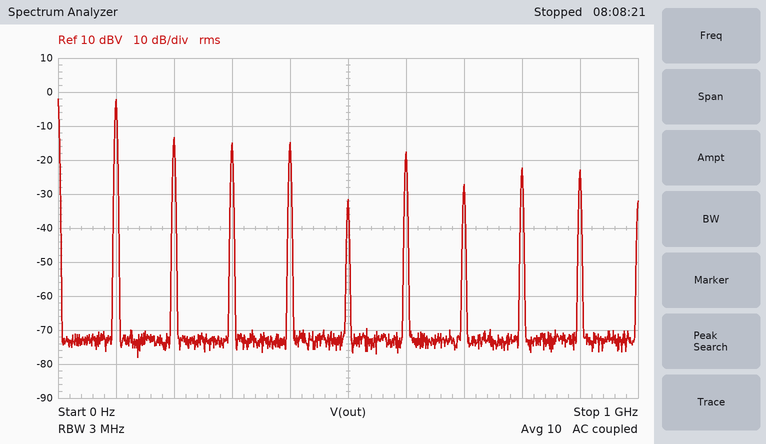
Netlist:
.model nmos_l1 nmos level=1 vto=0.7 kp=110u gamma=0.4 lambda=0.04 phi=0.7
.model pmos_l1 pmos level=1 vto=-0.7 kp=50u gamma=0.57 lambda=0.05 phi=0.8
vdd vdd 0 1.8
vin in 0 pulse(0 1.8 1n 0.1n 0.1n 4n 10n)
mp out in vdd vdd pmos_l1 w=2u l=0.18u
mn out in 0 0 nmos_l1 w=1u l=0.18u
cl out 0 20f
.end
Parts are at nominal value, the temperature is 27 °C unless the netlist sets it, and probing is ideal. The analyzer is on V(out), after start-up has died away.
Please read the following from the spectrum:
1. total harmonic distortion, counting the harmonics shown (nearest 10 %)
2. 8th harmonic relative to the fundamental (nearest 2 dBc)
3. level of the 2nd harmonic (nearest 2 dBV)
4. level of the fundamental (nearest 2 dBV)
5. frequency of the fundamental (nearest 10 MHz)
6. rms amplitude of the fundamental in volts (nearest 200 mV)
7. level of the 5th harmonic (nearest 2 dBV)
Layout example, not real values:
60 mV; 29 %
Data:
50 %; -20 dBc; -14 dBV; -2 dBV; 100 MHz; 800 mV; -32 dBV
